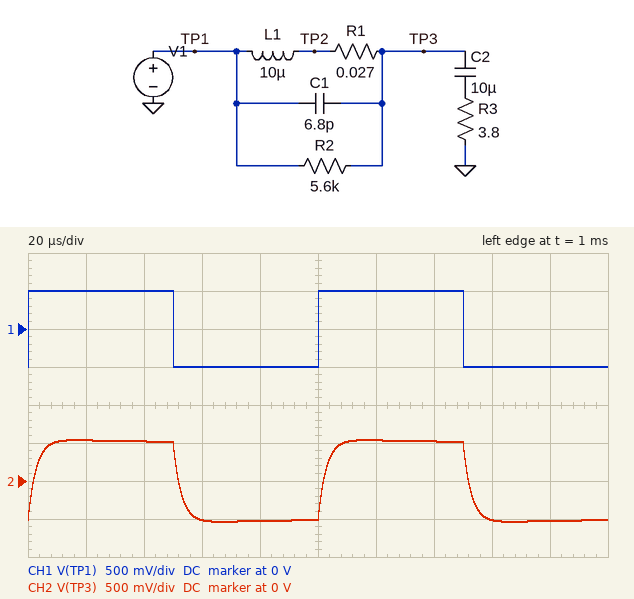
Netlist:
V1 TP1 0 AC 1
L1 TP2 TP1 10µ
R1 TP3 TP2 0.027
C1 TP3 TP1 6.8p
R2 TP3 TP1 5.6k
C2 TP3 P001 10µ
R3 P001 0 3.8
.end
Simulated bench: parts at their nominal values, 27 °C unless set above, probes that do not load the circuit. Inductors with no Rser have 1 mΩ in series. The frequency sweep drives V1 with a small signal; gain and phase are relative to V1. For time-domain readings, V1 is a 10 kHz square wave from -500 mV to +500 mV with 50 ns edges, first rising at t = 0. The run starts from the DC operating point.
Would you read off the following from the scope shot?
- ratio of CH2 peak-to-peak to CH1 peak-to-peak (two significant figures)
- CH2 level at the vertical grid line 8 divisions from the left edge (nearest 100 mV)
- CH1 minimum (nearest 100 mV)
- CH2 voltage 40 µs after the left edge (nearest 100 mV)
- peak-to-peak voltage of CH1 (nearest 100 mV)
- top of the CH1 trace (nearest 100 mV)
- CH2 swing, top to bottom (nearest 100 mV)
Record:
1.1
-500 mV
-500 mV
500 mV
1.0 V
500 mV
1.1 V
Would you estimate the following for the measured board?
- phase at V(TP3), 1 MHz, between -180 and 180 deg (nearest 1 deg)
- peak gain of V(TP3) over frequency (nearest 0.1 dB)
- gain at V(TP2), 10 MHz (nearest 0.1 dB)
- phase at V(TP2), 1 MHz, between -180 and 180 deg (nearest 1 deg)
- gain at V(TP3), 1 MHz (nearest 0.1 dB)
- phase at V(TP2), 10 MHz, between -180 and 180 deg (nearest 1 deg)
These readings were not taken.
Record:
-86 deg
0.4 dB
-46.9 dB
-86 deg
-24.4 dB
-81 deg
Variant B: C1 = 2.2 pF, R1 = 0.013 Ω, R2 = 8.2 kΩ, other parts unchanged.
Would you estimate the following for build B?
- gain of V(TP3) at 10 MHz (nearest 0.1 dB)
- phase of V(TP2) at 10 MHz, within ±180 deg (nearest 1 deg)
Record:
-45.1 dB
-85 deg
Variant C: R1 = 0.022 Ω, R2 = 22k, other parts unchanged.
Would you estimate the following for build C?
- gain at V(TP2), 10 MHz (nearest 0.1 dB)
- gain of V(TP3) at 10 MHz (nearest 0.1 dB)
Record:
-47.0 dB
-47.1 dB
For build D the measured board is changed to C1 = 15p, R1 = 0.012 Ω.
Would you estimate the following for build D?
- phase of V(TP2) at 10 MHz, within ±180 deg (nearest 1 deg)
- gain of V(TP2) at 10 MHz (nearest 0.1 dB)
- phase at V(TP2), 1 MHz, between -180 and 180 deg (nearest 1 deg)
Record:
-75 deg
-51.8 dB
-86 deg
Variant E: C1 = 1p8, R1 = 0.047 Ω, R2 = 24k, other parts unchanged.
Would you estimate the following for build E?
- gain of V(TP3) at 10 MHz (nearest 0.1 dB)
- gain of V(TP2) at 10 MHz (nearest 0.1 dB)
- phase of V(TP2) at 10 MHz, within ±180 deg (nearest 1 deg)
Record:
-45.0 dB
-44.9 dB
-88 deg
